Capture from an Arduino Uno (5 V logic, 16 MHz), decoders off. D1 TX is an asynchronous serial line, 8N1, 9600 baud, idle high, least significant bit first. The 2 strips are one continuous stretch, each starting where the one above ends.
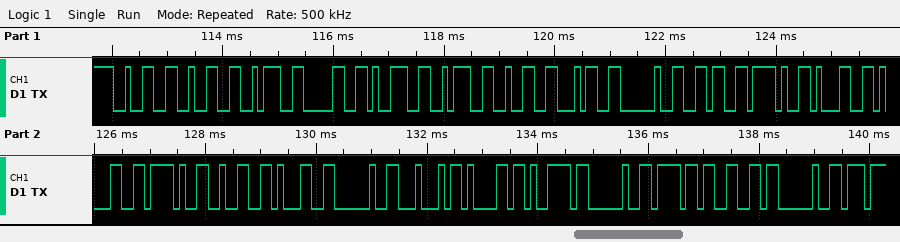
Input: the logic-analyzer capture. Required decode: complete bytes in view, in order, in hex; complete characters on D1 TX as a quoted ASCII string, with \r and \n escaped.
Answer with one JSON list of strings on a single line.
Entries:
["0x32 0x32 0x3A 0x30 0x39 0x3A 0x32 0x34 0x20 0x36 0x2F 0x31 0x31 0x2F 0x32 0x31 0x20 0x44 0x61 0x79 0x20 0x6F 0x66 0x20", "\"22:09:24 6/11/21 Day of \""]
